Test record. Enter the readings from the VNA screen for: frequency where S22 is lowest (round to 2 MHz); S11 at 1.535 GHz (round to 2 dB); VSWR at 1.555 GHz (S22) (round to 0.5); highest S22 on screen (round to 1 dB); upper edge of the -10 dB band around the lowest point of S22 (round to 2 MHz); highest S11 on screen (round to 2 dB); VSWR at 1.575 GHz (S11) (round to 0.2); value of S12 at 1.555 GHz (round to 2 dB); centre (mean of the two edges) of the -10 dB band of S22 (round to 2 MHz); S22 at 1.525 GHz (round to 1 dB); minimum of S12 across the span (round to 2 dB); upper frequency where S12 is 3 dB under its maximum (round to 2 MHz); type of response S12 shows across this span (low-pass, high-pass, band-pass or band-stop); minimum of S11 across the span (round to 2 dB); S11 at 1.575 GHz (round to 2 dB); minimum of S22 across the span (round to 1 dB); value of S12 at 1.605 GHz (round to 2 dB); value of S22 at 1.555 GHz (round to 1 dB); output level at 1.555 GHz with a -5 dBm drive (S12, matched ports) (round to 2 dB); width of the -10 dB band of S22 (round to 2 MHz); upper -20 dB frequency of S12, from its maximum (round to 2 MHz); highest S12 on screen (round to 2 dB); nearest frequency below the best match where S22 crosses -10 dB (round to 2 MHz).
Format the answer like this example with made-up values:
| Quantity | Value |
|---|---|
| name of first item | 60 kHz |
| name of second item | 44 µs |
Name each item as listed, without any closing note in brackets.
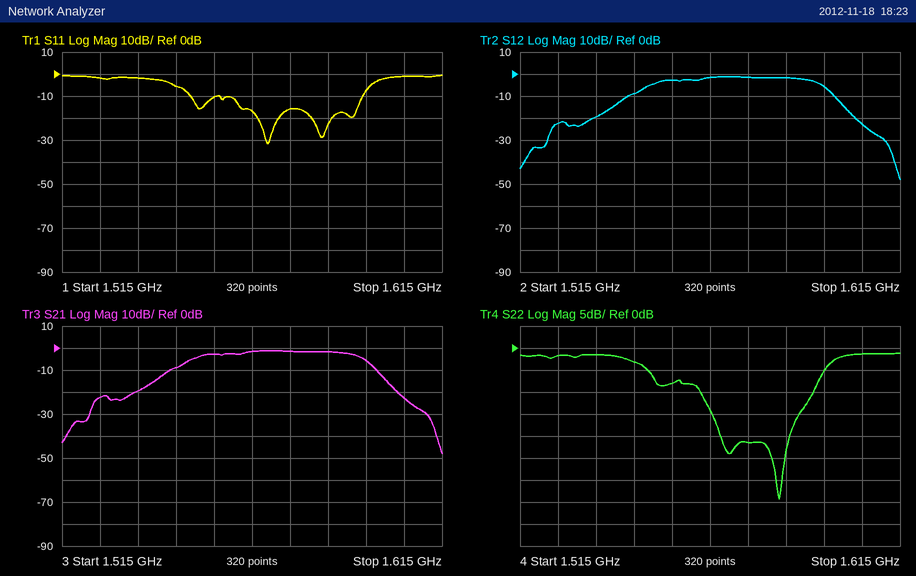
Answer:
| Quantity | Value |
|---|---|
| frequency where S22 is lowest | 1.584 GHz |
| S11 at 1.535 GHz | -2 dB |
| VSWR at 1.555 GHz (S22) | 2.5 |
| highest S22 on screen | -1 dB |
| upper edge of the -10 dB band around the lowest point of S22 | 1.592 GHz |
| highest S11 on screen | 0 dB |
| VSWR at 1.575 GHz (S11) | 1.4 |
| value of S12 at 1.555 GHz | -2 dB |
| centre (mean of the two edges) of the -10 dB band of S22 | 1.578 GHz |
| S22 at 1.525 GHz | -2 dB |
| minimum of S12 across the span | -48 dB |
| upper frequency where S12 is 3 dB under its maximum | 1.594 GHz |
| type of response S12 shows across this span | band-pass |
| minimum of S11 across the span | -32 dB |
| S11 at 1.575 GHz | -16 dB |
| minimum of S22 across the span | -34 dB |
| value of S12 at 1.605 GHz | -22 dB |
| value of S22 at 1.555 GHz | -8 dB |
| output level at 1.555 GHz with a -5 dBm drive (S12, matched ports) | -8 dBm |
| width of the -10 dB band of S22 | 30 MHz |
| upper -20 dB frequency of S12, from its maximum | 1.604 GHz |
| highest S12 on screen | -2 dB |
| nearest frequency below the best match where S22 crosses -10 dB | 1.562 GHz |
